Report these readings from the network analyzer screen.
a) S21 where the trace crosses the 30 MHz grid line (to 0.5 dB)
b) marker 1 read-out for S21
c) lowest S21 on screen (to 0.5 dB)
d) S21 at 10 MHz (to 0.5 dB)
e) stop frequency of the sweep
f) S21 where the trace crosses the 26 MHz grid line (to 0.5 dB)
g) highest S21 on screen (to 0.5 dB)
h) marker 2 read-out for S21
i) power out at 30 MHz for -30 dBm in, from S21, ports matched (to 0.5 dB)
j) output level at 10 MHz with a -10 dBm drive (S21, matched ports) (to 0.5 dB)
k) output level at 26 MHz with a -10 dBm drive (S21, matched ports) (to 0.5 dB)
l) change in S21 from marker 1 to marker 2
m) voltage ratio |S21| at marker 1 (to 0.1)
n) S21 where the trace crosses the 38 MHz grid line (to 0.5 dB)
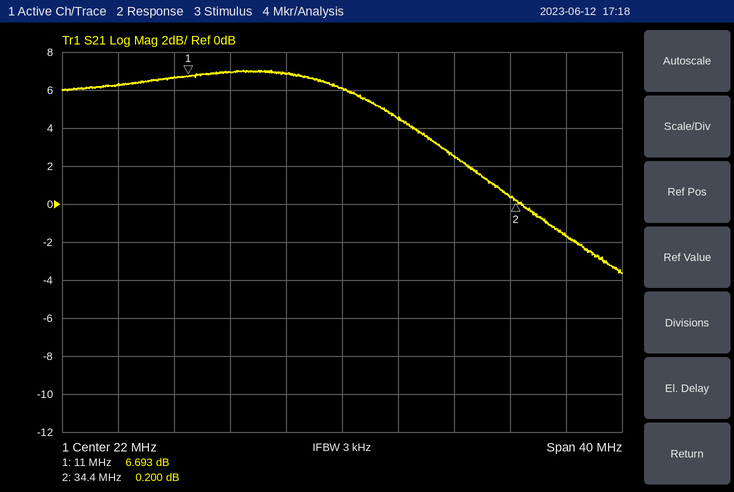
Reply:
2.5 dB
6.693 dB
-3.5 dB
6.5 dB
42 MHz
4.5 dB
7.0 dB
0.200 dB
-27.5 dBm
-3.5 dBm
-5.5 dBm
-6.493 dB
2.2
-1.5 dB
